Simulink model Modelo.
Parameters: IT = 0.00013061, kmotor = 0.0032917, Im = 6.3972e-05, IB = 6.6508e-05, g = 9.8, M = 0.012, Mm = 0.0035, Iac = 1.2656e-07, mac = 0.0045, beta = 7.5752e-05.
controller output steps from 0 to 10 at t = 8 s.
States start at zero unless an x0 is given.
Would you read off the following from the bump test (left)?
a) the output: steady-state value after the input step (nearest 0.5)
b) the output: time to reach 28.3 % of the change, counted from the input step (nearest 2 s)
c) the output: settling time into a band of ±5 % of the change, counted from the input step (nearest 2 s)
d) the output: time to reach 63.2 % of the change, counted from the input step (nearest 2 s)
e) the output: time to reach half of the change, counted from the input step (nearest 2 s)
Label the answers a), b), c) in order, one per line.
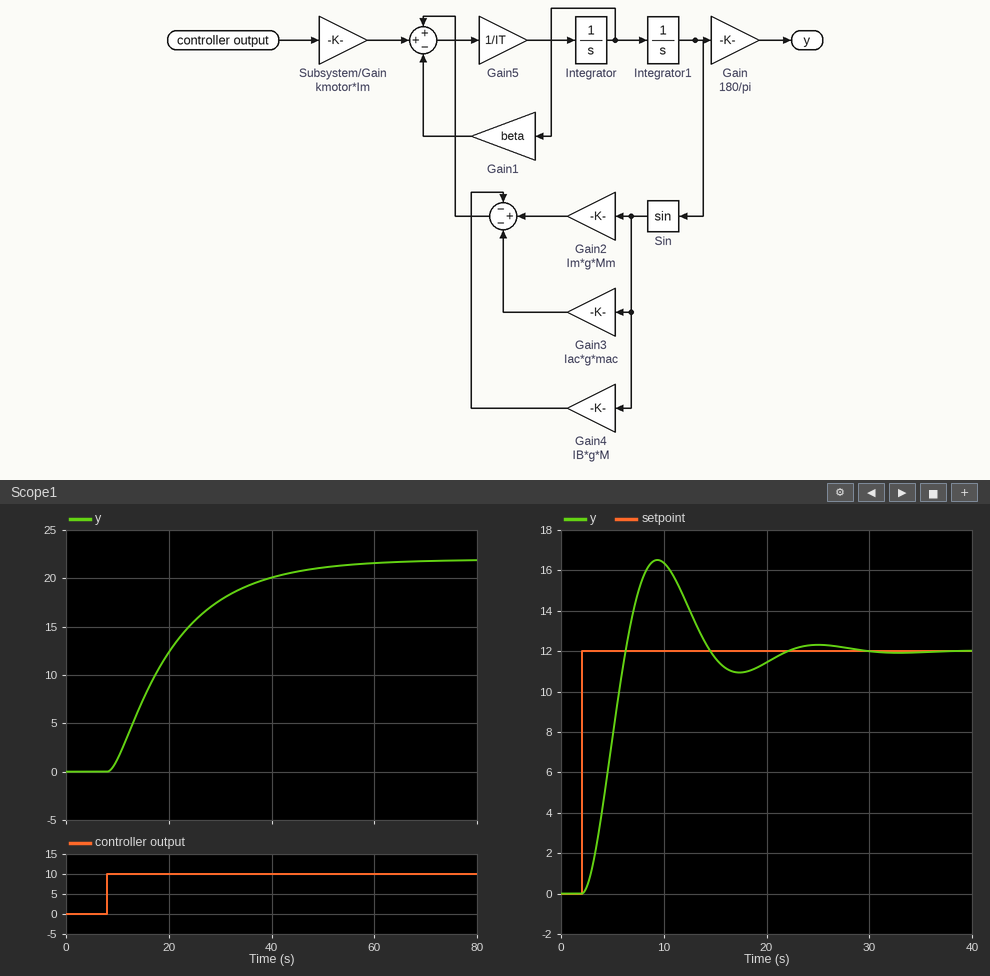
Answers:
a) 22.0
b) 6 s
c) 38 s
d) 14 s
e) 10 s
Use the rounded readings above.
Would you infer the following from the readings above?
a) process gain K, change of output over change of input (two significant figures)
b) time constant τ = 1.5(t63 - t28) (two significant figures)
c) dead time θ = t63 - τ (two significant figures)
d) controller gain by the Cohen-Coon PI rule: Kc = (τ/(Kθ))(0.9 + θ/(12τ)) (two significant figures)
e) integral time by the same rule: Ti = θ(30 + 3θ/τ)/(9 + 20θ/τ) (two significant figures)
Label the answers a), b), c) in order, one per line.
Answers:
a) 2.2
b) 12 s
c) 2.0 s
d) 2.5
e) 4.9 s
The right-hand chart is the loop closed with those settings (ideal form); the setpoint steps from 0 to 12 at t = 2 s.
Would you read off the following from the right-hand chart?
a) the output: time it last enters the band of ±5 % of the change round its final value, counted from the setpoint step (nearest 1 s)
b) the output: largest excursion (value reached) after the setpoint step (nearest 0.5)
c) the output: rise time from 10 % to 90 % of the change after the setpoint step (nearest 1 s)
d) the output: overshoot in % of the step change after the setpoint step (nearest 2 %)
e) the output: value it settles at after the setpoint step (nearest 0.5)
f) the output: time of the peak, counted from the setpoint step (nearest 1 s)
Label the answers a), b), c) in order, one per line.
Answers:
a) 18 s
b) 16.5
c) 3 s
d) 38 %
e) 12.0
f) 7 s
